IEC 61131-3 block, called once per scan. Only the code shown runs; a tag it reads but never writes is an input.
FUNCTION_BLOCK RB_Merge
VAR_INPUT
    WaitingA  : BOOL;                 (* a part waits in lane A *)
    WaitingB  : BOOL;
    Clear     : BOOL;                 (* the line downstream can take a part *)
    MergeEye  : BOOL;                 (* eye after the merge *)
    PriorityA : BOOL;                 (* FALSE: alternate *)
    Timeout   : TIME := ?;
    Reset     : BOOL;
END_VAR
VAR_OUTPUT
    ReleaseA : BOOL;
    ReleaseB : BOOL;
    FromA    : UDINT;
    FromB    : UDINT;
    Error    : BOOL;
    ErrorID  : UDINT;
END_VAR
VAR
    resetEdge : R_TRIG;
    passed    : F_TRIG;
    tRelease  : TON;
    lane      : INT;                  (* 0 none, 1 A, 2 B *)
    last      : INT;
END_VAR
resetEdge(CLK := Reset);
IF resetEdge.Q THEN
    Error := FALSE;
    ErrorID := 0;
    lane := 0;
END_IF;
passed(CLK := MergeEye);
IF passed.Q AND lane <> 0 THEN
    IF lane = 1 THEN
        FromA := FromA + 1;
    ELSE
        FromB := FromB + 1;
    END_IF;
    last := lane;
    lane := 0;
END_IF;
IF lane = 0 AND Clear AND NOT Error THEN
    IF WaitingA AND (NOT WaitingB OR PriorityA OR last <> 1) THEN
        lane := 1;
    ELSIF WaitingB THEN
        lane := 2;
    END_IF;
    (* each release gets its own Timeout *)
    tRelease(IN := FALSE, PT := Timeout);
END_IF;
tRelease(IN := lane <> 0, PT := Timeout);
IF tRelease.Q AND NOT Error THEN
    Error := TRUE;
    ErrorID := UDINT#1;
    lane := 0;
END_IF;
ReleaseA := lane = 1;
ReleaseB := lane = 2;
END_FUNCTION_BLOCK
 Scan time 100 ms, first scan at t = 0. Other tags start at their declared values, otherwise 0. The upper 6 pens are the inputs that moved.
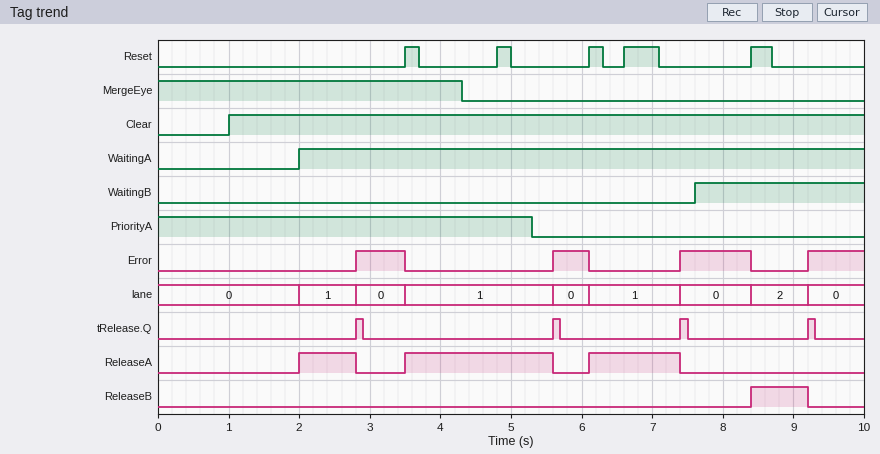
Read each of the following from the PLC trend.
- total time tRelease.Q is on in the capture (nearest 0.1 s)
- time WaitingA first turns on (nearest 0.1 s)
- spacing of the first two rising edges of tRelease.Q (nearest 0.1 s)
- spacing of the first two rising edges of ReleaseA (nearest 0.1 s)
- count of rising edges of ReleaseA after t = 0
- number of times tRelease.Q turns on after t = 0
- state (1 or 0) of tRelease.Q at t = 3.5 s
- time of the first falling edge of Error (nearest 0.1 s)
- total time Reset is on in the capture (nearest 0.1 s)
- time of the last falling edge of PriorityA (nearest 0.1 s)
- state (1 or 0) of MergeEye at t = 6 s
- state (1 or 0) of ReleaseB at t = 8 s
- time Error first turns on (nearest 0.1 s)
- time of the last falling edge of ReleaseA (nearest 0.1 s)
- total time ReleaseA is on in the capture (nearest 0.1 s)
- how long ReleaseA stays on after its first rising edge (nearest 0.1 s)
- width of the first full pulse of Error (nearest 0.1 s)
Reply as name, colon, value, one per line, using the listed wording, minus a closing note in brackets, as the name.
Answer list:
total time tRelease.Q is on in the capture: 0.4 s
time WaitingA first turns on: 2.0 s
spacing of the first two rising edges of tRelease.Q: 2.8 s
spacing of the first two rising edges of ReleaseA: 1.5 s
count of rising edges of ReleaseA after t = 0: 3
number of times tRelease.Q turns on after t = 0: 4
state (1 or 0) of tRelease.Q at t = 3.5 s: 0
time of the first falling edge of Error: 3.5 s
total time Reset is on in the capture: 1.4 s
time of the last falling edge of PriorityA: 5.3 s
state (1 or 0) of MergeEye at t = 6 s: 0
state (1 or 0) of ReleaseB at t = 8 s: 0
time Error first turns on: 2.8 s
time of the last falling edge of ReleaseA: 7.4 s
total time ReleaseA is on in the capture: 4.2 s
how long ReleaseA stays on after its first rising edge: 0.8 s
width of the first full pulse of Error: 0.7 s
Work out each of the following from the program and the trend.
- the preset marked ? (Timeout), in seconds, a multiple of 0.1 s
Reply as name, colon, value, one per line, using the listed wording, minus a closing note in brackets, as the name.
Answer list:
the preset marked ? (Timeout), in seconds, a multiple of 0.1 s: 0.8 s
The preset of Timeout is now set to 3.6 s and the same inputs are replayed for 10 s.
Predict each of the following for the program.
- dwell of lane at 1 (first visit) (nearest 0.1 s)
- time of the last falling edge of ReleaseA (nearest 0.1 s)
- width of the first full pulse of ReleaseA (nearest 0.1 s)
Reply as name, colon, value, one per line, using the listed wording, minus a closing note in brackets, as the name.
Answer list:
dwell of lane at 1 (first visit): 6.4 s
time of the last falling edge of ReleaseA: 8.4 s
width of the first full pulse of ReleaseA: 6.4 s
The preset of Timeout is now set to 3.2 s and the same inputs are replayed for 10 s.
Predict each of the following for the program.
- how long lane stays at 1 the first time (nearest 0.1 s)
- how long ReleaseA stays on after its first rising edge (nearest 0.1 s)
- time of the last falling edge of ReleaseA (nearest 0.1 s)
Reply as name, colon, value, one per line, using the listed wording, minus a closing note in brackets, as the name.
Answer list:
how long lane stays at 1 the first time: 6.4 s
how long ReleaseA stays on after its first rising edge: 6.4 s
time of the last falling edge of ReleaseA: 8.4 s
